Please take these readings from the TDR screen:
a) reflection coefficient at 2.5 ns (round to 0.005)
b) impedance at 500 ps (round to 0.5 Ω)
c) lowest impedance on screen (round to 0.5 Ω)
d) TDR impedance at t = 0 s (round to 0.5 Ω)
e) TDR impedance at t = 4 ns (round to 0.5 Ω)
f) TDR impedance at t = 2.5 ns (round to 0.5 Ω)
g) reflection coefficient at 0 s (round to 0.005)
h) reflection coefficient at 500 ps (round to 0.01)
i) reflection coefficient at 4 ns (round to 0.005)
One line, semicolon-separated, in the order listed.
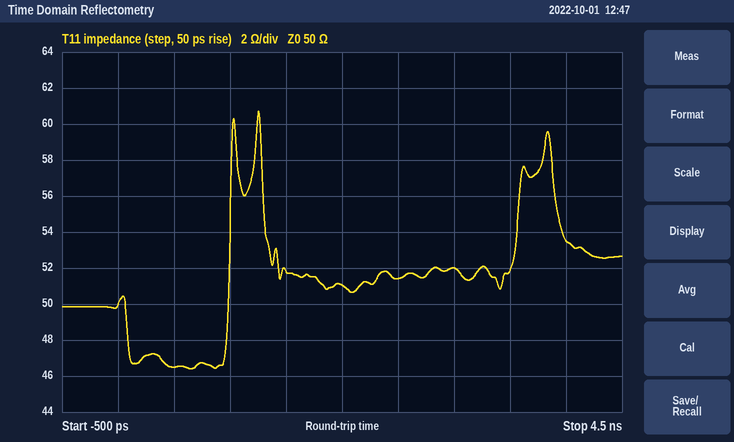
+0.015; 46.5 Ω; 46.5 Ω; 50.0 Ω; 53.5 Ω; 51.5 Ω; 0.000; -0.04; +0.035
